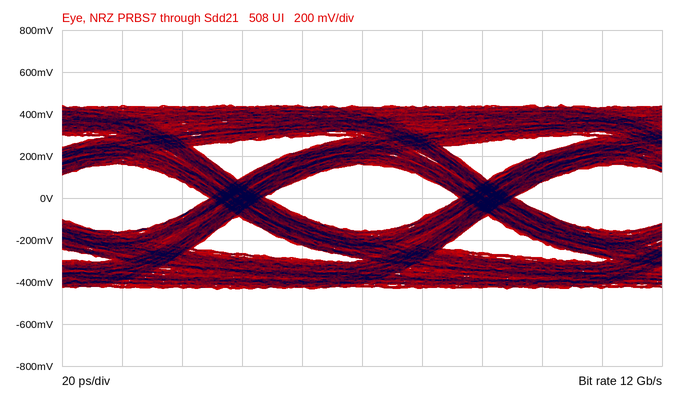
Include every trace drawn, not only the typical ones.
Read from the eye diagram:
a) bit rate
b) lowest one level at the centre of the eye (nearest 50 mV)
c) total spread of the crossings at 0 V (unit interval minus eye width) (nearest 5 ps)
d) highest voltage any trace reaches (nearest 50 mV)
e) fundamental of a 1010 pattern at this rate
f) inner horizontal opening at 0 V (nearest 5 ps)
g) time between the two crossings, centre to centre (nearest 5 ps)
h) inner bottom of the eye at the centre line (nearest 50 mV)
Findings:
12 Gb/s
150 mV
20 ps
450 mV
6 GHz
65 ps
85 ps
-150 mV
